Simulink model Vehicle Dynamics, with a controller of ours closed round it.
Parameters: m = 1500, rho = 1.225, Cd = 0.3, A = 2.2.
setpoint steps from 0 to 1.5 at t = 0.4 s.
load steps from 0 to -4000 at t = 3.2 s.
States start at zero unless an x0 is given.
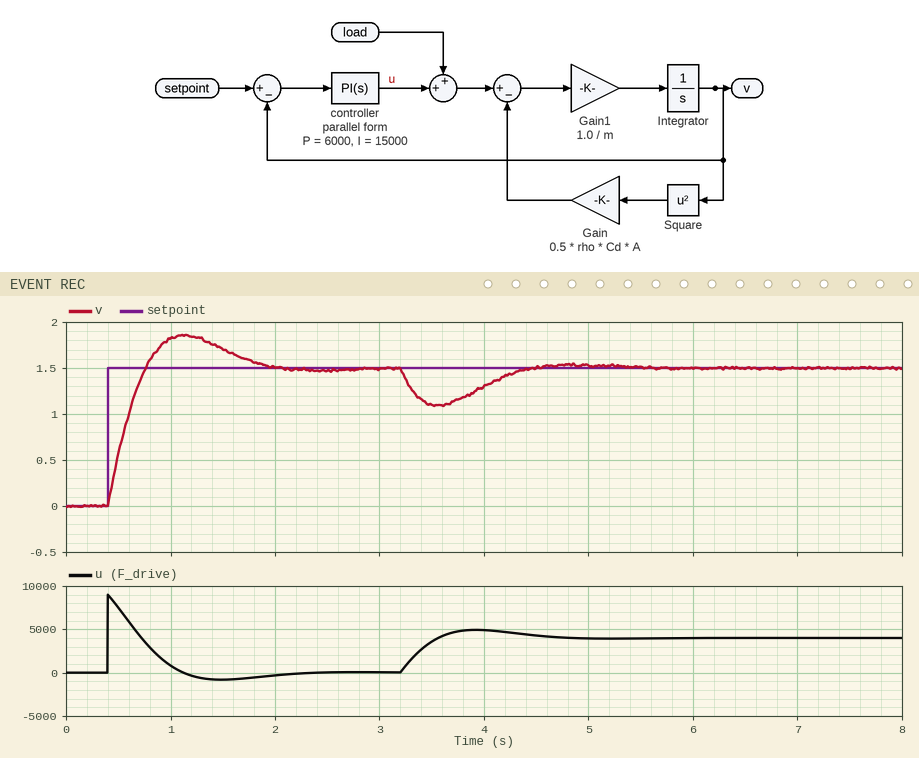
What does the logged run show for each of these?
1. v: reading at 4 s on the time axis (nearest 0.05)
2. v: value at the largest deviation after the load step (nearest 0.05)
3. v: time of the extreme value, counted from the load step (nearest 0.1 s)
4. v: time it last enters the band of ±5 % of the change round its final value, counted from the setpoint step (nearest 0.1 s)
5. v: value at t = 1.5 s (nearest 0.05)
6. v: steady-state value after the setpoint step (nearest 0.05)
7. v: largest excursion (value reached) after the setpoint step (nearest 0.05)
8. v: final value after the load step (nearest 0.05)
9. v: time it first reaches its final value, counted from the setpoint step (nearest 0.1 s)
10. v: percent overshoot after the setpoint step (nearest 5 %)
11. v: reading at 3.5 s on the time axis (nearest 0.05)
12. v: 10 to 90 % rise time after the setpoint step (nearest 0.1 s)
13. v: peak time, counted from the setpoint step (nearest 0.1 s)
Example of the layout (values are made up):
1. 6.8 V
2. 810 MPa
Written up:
1. 1.30
2. 1.10
3. 0.4 s
4. 1.4 s
5. 1.70
6. 1.50
7. 1.85
8. 1.50
9. 0.4 s
10. 25 %
11. 1.10
12. 0.3 s
13. 0.7 s
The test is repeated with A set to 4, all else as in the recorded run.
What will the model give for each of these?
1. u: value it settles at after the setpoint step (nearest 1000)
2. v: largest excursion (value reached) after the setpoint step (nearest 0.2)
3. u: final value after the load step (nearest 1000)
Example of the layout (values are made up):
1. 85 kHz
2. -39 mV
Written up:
1. 0
2. 1.8
3. 4000
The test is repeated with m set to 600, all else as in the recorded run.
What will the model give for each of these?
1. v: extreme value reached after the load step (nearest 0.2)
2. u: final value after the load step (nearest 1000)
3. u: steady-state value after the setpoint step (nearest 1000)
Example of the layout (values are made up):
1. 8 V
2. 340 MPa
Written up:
1. 1.0
2. 4000
3. 0
